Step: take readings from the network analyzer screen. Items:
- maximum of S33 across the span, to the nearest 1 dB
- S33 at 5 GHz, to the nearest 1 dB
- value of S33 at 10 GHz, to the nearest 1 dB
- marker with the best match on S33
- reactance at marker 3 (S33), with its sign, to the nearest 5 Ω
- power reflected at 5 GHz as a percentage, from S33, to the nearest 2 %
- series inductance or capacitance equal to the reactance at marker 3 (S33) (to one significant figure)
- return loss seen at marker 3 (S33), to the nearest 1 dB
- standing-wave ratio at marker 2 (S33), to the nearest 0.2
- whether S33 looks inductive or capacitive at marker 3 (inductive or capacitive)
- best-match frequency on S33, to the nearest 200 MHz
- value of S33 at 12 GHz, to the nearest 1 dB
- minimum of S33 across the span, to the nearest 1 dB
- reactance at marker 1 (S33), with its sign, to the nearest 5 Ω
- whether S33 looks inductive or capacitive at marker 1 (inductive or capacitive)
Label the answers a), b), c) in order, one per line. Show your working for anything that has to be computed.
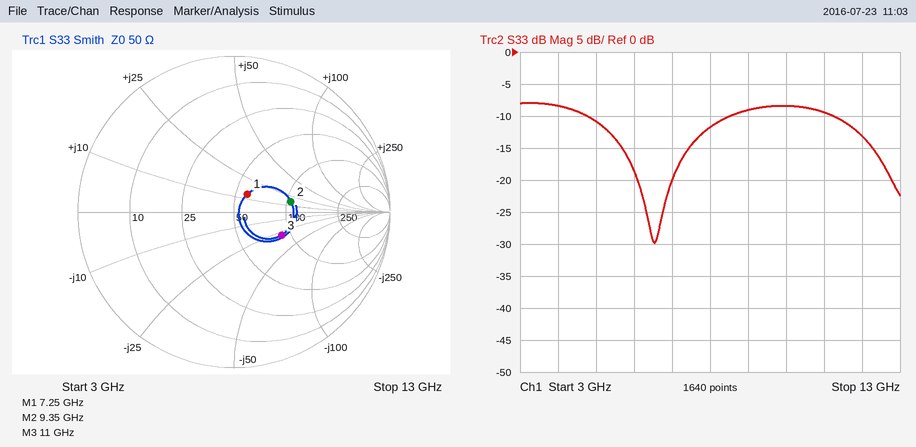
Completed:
a) -8 dB
b) -11 dB
c) -8 dB
d) marker 1
e) -30 Ω
f) 10^(-11/10) ≈ 8 %
g) C = 1/(2π × 11 GHz × 30 Ω) ≈ 482 fF, so 500 fF to one significant figure
h) 9 dB
i) 2.2
j) capacitive
k) 6.6 GHz
l) -13 dB
m) -30 dB
n) +15 Ω
o) inductive
